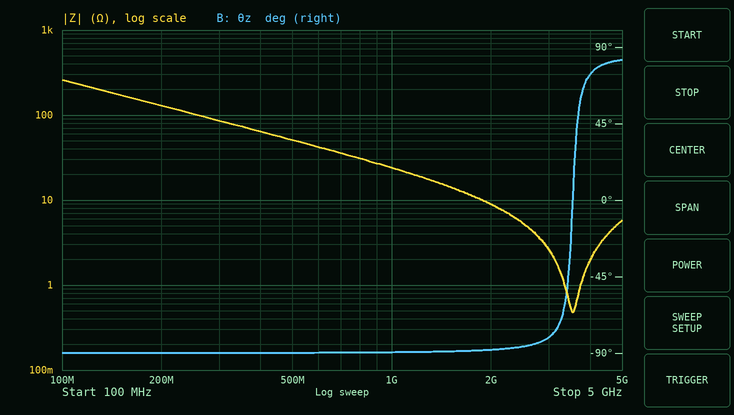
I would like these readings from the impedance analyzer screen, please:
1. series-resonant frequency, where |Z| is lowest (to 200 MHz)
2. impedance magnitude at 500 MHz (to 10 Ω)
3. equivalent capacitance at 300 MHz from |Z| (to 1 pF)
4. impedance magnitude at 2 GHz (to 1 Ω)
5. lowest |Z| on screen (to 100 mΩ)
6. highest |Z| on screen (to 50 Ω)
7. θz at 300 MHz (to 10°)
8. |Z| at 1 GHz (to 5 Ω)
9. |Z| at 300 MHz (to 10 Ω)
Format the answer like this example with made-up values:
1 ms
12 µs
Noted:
3.6 GHz
50 Ω
6 pF
9 Ω
500 mΩ
250 Ω
-90°
25 Ω
90 Ω
